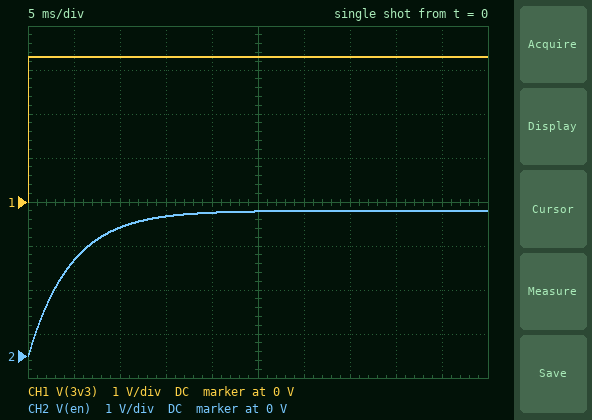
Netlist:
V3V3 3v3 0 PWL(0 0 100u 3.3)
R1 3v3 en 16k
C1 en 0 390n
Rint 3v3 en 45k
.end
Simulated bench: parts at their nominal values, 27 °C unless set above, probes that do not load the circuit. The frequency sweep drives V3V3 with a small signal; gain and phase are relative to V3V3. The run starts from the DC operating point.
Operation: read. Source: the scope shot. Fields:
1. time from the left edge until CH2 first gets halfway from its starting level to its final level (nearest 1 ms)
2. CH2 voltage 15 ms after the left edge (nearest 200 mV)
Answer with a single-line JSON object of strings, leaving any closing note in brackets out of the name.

{"time from the left edge until CH2 first gets halfway from its starting level to its final level": "3 ms", "CH2 voltage 15 ms after the left edge": "3.2 V"}
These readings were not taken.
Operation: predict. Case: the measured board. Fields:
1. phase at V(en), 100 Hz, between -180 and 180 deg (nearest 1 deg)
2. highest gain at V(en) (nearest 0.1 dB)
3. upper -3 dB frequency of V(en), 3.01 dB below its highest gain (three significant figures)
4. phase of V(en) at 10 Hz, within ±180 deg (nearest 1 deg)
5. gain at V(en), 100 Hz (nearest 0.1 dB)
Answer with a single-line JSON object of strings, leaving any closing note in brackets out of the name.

{"phase at V(en), 100 Hz, between -180 and 180 deg": "-71 deg", "highest gain at V(en)": "0 dB", "upper -3 dB frequency of V(en), 3.01 dB below its highest gain": "34.6 Hz", "phase of V(en) at 10 Hz, within ±180 deg": "-16 deg", "gain at V(en), 100 Hz": "-9.7 dB"}
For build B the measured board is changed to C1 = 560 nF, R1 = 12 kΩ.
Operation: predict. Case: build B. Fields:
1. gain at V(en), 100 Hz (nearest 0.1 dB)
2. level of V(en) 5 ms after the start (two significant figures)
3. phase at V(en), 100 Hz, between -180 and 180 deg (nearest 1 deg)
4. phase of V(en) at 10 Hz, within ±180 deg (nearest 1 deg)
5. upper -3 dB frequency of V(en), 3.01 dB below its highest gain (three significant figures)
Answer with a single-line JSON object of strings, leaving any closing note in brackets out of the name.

{"gain at V(en), 100 Hz": "-10.8 dB", "level of V(en) 5 ms after the start": "2.0 V", "phase at V(en), 100 Hz, between -180 and 180 deg": "-73 deg", "phase of V(en) at 10 Hz, within ±180 deg": "-18 deg", "upper -3 dB frequency of V(en), 3.01 dB below its highest gain": "30.0 Hz"}
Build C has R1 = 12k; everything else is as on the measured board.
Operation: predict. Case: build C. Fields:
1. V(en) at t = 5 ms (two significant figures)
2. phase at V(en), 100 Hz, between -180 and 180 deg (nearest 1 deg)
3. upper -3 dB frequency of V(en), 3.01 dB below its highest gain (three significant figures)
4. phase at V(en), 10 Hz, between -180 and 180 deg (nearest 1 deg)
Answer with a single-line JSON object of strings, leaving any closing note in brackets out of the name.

{"V(en) at t = 5 ms": "2.4 V", "phase at V(en), 100 Hz, between -180 and 180 deg": "-67 deg", "upper -3 dB frequency of V(en), 3.01 dB below its highest gain": "43.1 Hz", "phase at V(en), 10 Hz, between -180 and 180 deg": "-13 deg"}
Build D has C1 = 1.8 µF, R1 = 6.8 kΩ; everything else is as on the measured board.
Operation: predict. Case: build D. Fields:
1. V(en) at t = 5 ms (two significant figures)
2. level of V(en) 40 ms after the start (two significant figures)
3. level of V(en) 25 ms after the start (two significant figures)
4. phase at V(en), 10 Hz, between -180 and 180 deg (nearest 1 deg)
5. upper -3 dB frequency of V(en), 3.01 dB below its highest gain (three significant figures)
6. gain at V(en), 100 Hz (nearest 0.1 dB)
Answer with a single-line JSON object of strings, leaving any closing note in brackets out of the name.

{"V(en) at t = 5 ms": "1.2 V", "level of V(en) 40 ms after the start": "3.2 V", "level of V(en) 25 ms after the start": "3.0 V", "phase at V(en), 10 Hz, between -180 and 180 deg": "-34 deg", "upper -3 dB frequency of V(en), 3.01 dB below its highest gain": "15.0 Hz", "gain at V(en), 100 Hz": "-16.6 dB"}
